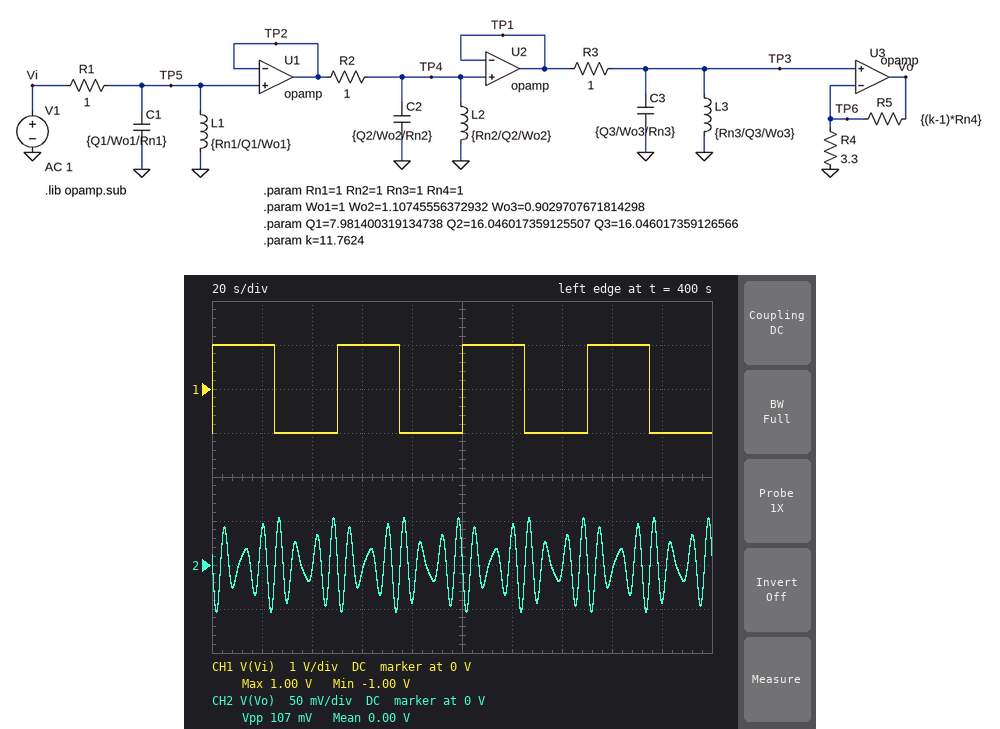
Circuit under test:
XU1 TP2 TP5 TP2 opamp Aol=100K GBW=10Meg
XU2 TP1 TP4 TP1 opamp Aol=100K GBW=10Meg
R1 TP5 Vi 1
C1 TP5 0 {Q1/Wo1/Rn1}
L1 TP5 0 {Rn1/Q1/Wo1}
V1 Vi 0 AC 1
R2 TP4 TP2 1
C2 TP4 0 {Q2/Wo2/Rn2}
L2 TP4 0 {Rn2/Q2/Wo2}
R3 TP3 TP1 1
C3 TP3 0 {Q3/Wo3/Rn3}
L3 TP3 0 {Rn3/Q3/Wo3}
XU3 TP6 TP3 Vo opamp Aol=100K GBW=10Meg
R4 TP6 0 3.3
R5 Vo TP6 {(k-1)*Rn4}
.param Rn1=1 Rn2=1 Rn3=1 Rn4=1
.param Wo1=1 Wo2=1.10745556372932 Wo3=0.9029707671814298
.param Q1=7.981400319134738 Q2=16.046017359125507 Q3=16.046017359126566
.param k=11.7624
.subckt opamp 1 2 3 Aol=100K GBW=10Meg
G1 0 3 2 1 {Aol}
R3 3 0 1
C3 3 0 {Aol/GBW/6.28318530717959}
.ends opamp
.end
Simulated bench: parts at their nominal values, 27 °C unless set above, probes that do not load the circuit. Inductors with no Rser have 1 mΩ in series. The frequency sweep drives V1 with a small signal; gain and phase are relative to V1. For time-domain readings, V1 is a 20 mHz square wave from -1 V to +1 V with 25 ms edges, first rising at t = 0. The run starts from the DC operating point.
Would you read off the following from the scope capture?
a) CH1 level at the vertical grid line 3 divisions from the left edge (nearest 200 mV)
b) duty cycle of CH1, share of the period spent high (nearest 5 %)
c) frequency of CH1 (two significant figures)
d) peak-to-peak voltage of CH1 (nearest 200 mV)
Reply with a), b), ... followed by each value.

a) 1.0 V
b) 50 %
c) 20 mHz
d) 2.0 V
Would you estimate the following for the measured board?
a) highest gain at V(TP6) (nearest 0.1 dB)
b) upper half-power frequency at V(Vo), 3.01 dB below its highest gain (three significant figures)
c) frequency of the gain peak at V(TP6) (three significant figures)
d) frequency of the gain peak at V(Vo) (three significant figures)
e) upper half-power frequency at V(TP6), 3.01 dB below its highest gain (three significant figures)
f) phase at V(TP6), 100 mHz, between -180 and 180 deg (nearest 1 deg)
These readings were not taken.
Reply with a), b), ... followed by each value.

a) -22.4 dB
b) 178 mHz
c) 159 mHz
d) 159 mHz
e) 178 mHz
f) -111 deg
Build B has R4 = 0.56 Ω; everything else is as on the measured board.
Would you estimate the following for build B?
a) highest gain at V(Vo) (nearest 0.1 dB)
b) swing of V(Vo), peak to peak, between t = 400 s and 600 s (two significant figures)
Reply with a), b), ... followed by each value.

a) 3.7 dB
b) 510 mV
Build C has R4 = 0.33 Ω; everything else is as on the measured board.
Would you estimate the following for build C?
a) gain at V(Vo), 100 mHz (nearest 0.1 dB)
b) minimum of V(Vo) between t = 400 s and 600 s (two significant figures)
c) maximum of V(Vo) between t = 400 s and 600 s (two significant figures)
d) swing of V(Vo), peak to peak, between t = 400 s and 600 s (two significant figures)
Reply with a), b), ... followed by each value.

a) -34.5 dB
b) -420 mV
c) 420 mV
d) 850 mV
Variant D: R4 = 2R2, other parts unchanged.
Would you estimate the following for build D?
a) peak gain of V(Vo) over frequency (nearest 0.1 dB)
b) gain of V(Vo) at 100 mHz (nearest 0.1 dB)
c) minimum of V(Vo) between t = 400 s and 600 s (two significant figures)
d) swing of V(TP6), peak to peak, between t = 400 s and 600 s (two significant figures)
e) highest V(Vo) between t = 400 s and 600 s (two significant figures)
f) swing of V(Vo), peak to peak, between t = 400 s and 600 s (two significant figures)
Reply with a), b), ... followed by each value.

a) -7.0 dB
b) -49.7 dB
c) -74 mV
d) 25 mV
e) 74 mV
f) 150 mV
